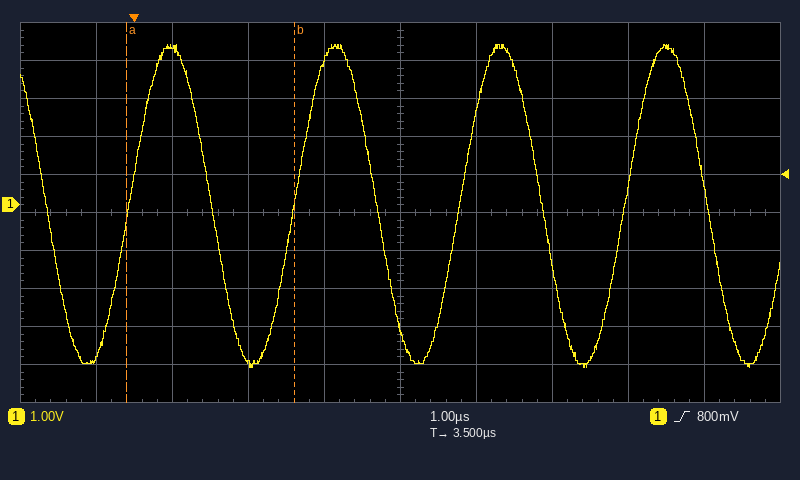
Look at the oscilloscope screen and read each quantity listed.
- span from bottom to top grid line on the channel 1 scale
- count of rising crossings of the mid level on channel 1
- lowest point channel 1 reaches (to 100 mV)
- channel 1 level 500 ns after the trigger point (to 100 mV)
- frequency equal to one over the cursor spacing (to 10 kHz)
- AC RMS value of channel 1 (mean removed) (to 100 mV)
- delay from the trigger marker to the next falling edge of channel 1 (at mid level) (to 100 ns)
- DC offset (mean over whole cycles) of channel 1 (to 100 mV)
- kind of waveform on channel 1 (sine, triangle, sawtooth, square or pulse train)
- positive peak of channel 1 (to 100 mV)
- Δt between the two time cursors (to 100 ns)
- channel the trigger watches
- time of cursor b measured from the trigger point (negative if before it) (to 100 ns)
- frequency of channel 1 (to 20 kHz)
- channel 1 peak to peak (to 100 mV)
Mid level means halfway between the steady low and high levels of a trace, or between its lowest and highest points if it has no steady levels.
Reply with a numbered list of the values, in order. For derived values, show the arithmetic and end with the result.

1. 10 V
2. 4
3. -4.3 V
4. 4.1 V
5. 1 / 2.2 µs ≈ 450 kHz
6. 8.5 V / (2√2) ≈ 3.0 V
7. 1.0 µs
8. (4.2 V + (-4.3 V)) / 2 ≈ 0.0 V
9. sine
10. 4.2 V
11. 2.2 µs
12. channel 1
13. +2.1 µs
14. 460 kHz
15. 4.2 V − (-4.3 V) = 8.5 V
